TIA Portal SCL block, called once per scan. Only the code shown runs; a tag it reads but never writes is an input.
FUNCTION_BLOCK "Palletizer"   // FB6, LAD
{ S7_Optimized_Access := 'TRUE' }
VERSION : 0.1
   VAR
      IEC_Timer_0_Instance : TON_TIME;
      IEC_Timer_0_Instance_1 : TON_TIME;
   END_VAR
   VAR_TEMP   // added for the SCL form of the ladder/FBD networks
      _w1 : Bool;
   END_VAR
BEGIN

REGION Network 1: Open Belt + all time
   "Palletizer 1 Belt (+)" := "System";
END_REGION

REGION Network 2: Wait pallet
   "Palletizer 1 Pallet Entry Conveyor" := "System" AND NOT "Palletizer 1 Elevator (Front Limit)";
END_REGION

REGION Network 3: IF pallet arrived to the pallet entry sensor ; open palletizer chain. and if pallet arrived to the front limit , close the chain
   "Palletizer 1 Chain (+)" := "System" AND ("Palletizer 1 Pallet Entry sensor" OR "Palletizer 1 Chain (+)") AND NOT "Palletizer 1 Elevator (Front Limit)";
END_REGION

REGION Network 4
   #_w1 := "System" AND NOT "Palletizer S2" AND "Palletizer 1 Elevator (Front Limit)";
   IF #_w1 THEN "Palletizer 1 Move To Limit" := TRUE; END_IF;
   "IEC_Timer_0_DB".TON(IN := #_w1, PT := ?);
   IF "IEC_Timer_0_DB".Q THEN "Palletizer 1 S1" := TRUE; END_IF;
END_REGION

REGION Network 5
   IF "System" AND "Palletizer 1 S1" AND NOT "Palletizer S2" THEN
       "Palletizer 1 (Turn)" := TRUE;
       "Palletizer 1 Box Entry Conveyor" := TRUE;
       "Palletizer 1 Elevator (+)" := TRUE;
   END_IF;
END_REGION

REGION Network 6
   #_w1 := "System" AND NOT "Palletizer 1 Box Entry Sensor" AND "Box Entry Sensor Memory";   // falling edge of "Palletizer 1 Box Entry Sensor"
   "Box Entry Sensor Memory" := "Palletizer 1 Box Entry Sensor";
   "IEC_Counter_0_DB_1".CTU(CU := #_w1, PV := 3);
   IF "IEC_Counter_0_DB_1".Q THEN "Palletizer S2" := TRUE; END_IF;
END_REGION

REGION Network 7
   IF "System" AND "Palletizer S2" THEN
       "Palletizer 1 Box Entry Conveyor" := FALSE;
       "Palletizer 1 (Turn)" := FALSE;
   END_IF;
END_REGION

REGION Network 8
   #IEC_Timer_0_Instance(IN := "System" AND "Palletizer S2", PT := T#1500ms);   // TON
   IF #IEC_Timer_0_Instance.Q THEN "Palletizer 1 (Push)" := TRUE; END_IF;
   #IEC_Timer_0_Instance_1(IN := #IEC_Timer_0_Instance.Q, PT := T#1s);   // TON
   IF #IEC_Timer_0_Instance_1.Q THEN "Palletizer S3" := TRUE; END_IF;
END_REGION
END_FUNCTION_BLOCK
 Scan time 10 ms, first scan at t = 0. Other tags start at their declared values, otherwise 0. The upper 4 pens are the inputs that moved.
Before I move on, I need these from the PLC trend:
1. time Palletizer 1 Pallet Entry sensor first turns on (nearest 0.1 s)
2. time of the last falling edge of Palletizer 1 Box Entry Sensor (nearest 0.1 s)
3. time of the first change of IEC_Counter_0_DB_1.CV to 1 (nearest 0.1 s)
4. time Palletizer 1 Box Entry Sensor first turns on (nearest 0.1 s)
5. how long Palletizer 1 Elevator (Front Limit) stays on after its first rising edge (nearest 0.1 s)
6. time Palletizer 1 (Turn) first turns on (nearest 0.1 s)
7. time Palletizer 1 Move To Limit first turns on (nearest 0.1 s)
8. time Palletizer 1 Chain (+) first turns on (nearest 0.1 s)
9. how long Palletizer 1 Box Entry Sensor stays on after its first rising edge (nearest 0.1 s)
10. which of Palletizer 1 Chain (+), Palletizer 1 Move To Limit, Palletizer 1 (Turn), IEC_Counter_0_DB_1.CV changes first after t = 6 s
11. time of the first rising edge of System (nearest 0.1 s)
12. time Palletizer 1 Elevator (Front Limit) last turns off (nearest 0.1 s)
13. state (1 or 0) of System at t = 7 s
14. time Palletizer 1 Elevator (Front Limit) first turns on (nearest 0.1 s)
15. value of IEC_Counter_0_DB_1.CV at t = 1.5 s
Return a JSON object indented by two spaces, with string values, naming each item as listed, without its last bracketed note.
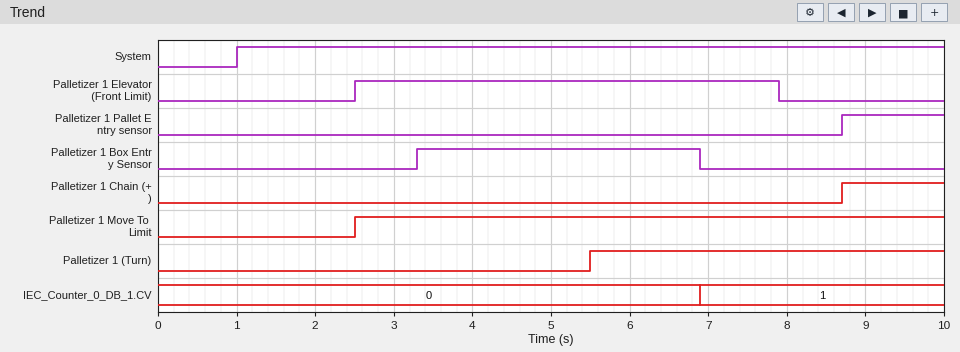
{
  "time Palletizer 1 Pallet Entry sensor first turns on": "8.7 s",
  "time of the last falling edge of Palletizer 1 Box Entry Sensor": "6.9 s",
  "time of the first change of IEC_Counter_0_DB_1.CV to 1": "6.9 s",
  "time Palletizer 1 Box Entry Sensor first turns on": "3.3 s",
  "how long Palletizer 1 Elevator (Front Limit) stays on after its first rising edge": "5.4 s",
  "time Palletizer 1 (Turn) first turns on": "5.5 s",
  "time Palletizer 1 Move To Limit first turns on": "2.5 s",
  "time Palletizer 1 Chain (+) first turns on": "8.7 s",
  "how long Palletizer 1 Box Entry Sensor stays on after its first rising edge": "3.6 s",
  "which of Palletizer 1 Chain (+), Palletizer 1 Move To Limit, Palletizer 1 (Turn), IEC_Counter_0_DB_1.CV changes first after t = 6 s": "IEC_Counter_0_DB_1.CV",
  "time of the first rising edge of System": "1.0 s",
  "time Palletizer 1 Elevator (Front Limit) last turns off": "7.9 s",
  "state (1 or 0) of System at t = 7 s": "1",
  "time Palletizer 1 Elevator (Front Limit) first turns on": "2.5 s",
  "value of IEC_Counter_0_DB_1.CV at t = 1.5 s": "0"
}
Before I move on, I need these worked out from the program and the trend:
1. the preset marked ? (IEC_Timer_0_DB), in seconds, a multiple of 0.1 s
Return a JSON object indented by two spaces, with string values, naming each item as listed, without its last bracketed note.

{
  "the preset marked ? (IEC_Timer_0_DB), in seconds, a multiple of 0.1 s": "3.0 s"
}
